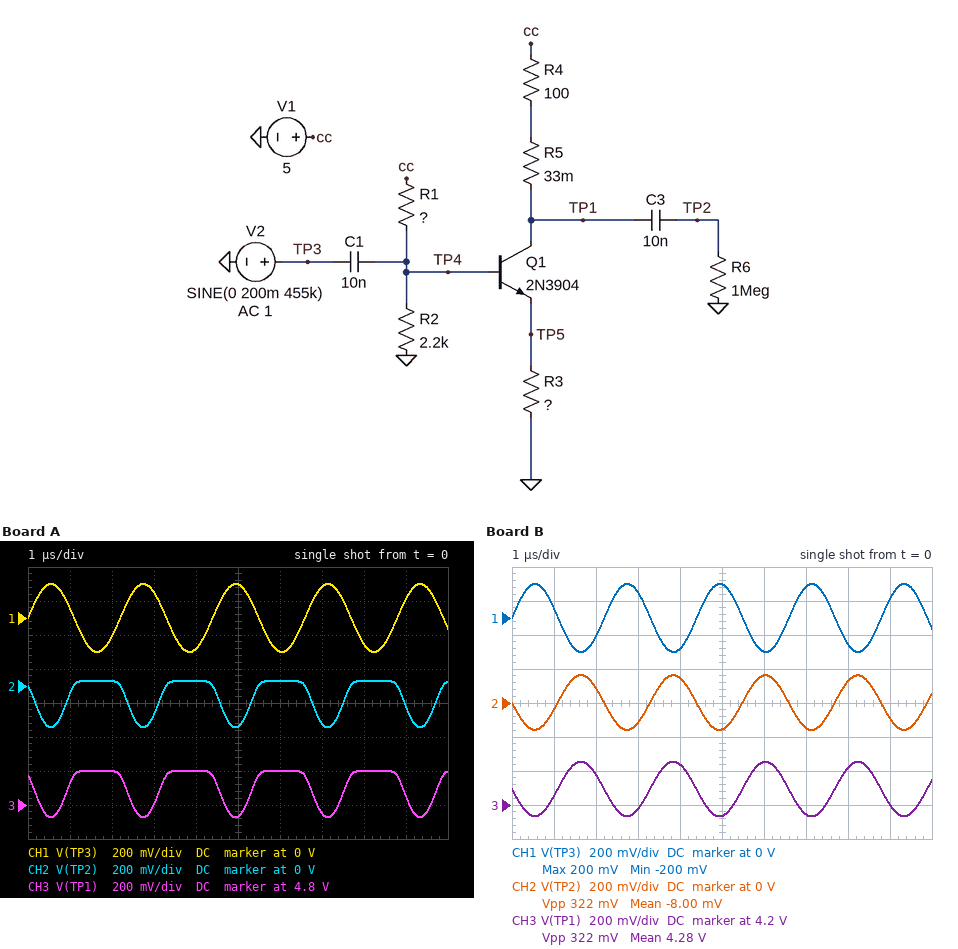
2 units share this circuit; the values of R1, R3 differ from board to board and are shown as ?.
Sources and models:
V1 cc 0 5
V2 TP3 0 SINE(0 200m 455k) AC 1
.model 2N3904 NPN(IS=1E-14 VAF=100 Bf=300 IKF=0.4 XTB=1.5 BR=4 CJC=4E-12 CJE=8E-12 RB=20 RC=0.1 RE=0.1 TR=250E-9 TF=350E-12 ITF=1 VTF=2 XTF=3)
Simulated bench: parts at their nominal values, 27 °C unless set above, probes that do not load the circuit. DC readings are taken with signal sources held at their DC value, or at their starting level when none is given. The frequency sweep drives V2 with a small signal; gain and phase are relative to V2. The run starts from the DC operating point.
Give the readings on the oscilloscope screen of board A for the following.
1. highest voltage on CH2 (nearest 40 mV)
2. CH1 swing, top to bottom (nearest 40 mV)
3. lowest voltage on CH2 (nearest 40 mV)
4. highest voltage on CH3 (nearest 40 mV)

40 mV
400 mV
-240 mV
5.00 V
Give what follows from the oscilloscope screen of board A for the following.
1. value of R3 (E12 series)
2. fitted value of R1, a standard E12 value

56 Ω
15 kΩ
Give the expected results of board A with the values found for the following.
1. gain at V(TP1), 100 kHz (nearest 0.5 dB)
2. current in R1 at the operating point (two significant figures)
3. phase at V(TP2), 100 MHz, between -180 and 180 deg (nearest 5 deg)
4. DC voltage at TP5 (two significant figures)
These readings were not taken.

-3.5 dB
290 µA
135 deg
16 mV
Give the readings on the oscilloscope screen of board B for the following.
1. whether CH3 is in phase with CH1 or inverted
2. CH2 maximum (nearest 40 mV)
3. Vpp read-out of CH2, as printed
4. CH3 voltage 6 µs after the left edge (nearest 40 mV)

inverted
160 mV
322 mV
4.44 V
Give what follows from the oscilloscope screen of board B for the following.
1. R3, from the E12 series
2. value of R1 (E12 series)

120 Ω
4.7 kΩ
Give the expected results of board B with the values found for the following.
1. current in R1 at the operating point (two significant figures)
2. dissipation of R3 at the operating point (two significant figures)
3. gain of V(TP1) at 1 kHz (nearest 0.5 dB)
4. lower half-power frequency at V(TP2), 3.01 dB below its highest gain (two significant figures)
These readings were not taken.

730 µA
6.1 mW
-23.0 dB
11 kHz
